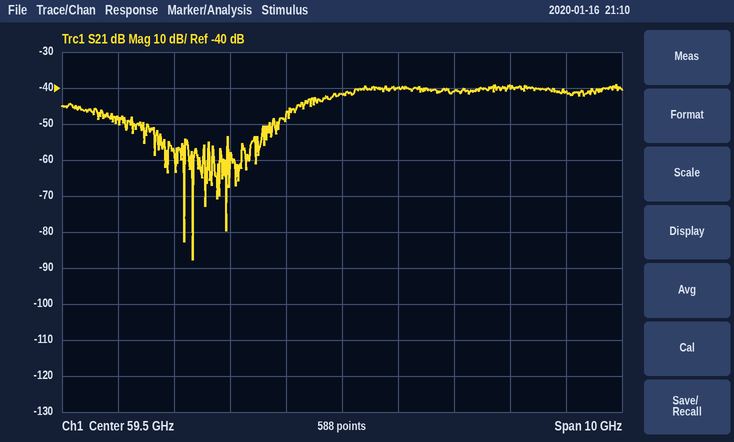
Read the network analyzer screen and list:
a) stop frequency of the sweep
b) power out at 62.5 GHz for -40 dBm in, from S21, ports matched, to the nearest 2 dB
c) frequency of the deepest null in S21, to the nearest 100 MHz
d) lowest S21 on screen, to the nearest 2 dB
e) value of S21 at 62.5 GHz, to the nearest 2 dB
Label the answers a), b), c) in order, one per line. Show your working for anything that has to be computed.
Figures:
a) 64.5 GHz
b) -40 dBm + (-40 dB) = -80 dBm
c) 56.8 GHz
d) -88 dB
e) -40 dB
